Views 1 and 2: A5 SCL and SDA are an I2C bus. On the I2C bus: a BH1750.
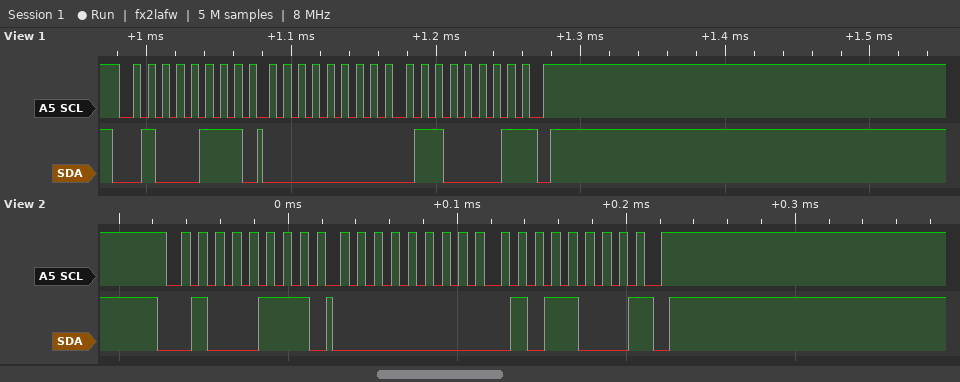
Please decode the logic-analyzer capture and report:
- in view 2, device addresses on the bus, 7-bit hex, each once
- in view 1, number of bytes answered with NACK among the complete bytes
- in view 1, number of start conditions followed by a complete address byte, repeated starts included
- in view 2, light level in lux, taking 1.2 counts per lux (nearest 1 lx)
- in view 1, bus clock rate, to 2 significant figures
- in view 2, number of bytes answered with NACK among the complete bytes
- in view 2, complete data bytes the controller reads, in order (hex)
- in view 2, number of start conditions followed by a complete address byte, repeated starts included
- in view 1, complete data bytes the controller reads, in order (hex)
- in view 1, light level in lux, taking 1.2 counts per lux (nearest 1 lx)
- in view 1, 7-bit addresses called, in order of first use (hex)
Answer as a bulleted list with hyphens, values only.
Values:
- 0x23
- 1
- 1
- 73 lx
- 100 kHz
- 1
- 00 58
- 1
- 00 61
- 81 lx
- 0x23
